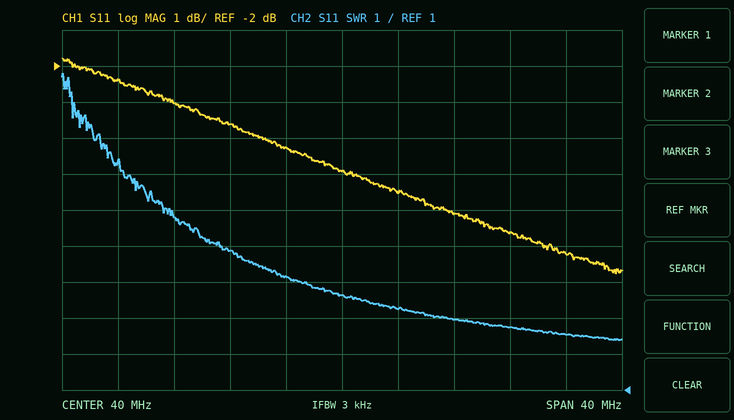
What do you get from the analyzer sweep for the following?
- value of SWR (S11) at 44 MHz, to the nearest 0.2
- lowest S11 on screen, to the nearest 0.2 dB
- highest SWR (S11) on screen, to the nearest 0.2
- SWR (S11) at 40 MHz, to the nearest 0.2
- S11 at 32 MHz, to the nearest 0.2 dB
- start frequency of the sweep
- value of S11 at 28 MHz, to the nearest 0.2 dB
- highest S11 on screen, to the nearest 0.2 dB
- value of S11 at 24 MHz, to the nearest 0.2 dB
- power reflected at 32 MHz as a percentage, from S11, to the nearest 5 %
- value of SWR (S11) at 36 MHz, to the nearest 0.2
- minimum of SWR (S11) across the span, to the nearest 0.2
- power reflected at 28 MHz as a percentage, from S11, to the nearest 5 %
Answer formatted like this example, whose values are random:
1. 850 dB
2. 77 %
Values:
1. 3.2
2. -7.8 dB
3. 9.8
4. 3.6
5. -3.6 dB
6. 20 MHz
7. -3.0 dB
8. -1.8 dB
9. -2.4 dB
10. 45 %
11. 4.2
12. 2.4
13. 50 %
